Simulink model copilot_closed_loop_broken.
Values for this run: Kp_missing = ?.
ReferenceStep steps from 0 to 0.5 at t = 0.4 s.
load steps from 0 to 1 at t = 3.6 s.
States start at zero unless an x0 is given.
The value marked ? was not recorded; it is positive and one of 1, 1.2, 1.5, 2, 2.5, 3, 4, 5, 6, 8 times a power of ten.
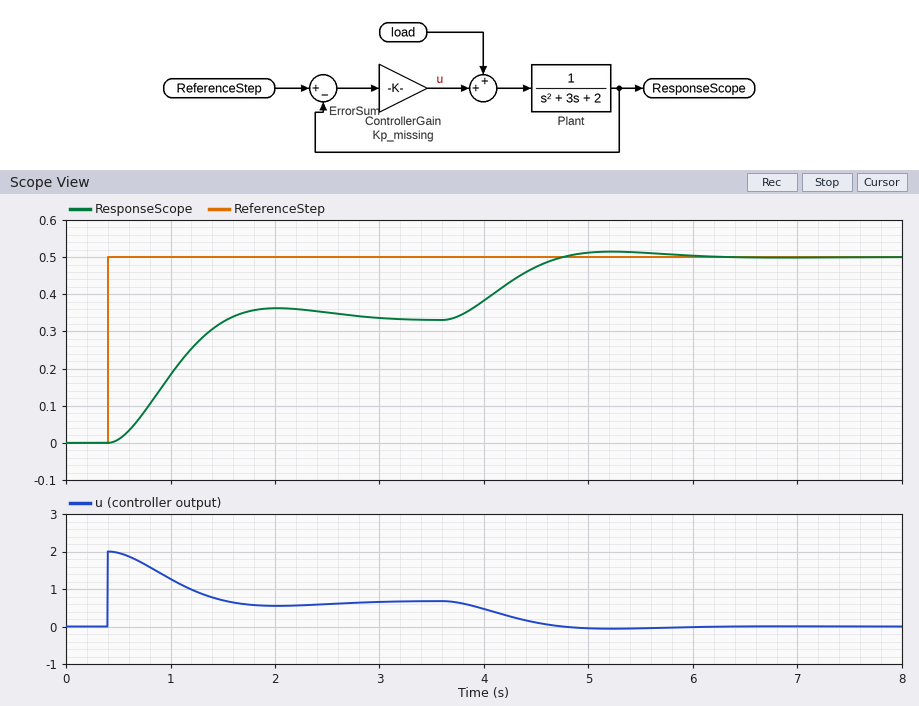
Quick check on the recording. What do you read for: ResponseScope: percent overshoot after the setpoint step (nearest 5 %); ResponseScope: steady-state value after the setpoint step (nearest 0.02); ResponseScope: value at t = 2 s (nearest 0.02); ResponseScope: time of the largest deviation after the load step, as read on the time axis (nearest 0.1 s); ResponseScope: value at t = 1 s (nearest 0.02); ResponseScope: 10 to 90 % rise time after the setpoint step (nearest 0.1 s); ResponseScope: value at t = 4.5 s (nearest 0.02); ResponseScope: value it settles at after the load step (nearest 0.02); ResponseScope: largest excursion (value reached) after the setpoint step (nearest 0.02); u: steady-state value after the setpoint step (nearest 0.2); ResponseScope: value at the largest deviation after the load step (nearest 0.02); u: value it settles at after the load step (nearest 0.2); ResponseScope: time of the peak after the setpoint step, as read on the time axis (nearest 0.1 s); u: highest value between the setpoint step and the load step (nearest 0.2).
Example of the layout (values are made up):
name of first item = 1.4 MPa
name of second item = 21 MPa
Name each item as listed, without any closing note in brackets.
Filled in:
ResponseScope: percent overshoot after the setpoint step = 10 %
ResponseScope: steady-state value after the setpoint step = 0.34
ResponseScope: value at t = 2 s = 0.36
ResponseScope: time of the largest deviation after the load step, as read on the time axis = 5.2 s
ResponseScope: value at t = 1 s = 0.18
ResponseScope: 10 to 90 % rise time after the setpoint step = 0.8 s
ResponseScope: value at t = 4.5 s = 0.48
ResponseScope: value it settles at after the load step = 0.50
ResponseScope: largest excursion (value reached) after the setpoint step = 0.36
u: steady-state value after the setpoint step = 0.6
ResponseScope: value at the largest deviation after the load step = 0.52
u: value it settles at after the load step = 0.0
ResponseScope: time of the peak after the setpoint step, as read on the time axis = 2.0 s
u: highest value between the setpoint step and the load step = 2.0
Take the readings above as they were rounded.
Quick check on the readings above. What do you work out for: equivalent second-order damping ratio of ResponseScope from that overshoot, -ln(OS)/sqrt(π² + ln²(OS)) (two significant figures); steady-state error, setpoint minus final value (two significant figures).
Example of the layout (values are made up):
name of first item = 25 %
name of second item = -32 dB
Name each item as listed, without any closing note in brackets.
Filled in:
equivalent second-order damping ratio of ResponseScope from that overshoot, -ln(OS)/sqrt(π² + ln²(OS)) = 0.59
steady-state error, setpoint minus final value = 0.16
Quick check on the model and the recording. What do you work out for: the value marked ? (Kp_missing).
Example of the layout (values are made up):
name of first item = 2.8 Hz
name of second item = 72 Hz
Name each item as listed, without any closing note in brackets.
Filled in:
the value marked ? = 4
